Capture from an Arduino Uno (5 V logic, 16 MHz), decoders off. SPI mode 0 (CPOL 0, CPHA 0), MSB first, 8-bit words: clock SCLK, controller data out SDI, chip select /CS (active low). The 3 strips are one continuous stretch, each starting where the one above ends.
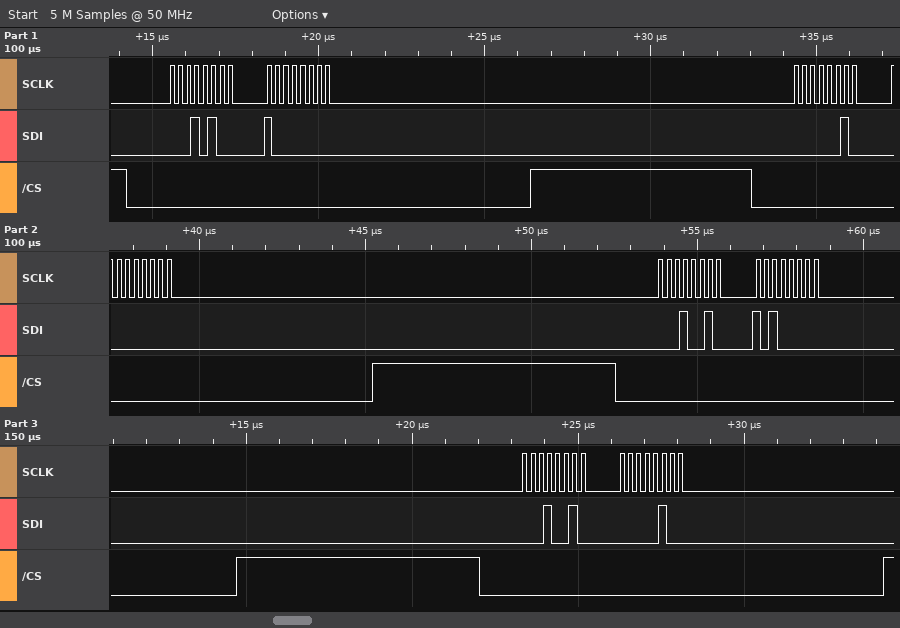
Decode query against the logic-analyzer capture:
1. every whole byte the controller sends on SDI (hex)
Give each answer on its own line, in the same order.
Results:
0x14 0x80 0x02 0x00 0x12 0xA0 0x12 0x04
